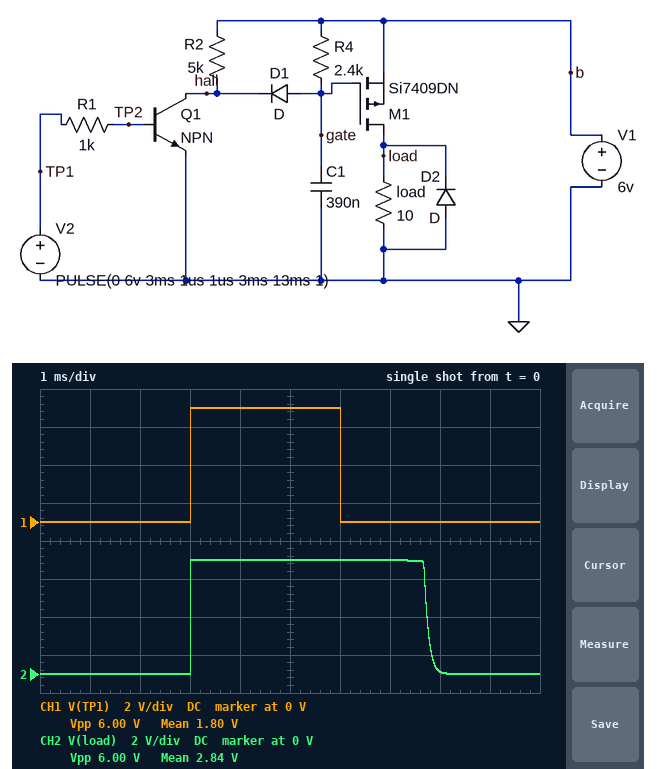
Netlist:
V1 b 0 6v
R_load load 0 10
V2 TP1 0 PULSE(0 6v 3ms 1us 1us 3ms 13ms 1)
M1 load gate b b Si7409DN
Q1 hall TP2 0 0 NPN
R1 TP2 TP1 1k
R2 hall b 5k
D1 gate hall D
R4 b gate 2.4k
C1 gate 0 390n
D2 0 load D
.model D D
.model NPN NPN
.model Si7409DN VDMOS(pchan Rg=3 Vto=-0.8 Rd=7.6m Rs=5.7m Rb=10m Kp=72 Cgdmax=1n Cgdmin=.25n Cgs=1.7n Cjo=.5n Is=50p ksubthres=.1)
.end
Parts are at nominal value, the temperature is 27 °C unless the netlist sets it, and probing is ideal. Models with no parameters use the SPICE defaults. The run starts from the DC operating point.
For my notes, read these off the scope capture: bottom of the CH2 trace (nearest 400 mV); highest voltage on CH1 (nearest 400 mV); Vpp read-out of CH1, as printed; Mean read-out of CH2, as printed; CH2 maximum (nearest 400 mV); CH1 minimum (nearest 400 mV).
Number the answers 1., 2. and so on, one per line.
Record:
1. 0 V
2. 6.0 V
3. 6.00 V
4. 2.84 V
5. 6.0 V
6. 0 V
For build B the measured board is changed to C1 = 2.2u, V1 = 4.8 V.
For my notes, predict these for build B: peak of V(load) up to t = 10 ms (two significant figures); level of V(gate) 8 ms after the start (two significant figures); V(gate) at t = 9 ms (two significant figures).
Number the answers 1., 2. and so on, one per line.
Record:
1. 4.8 V
2. 2.0 V
3. 2.5 V
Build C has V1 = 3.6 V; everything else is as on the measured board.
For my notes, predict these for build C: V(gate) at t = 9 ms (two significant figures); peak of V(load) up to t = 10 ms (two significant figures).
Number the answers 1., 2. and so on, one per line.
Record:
1. 3.5 V
2. 3.6 V
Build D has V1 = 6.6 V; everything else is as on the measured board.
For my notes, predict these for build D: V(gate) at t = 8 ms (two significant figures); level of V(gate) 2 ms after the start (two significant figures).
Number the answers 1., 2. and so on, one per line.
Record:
1. 5.9 V
2. 6.6 V
